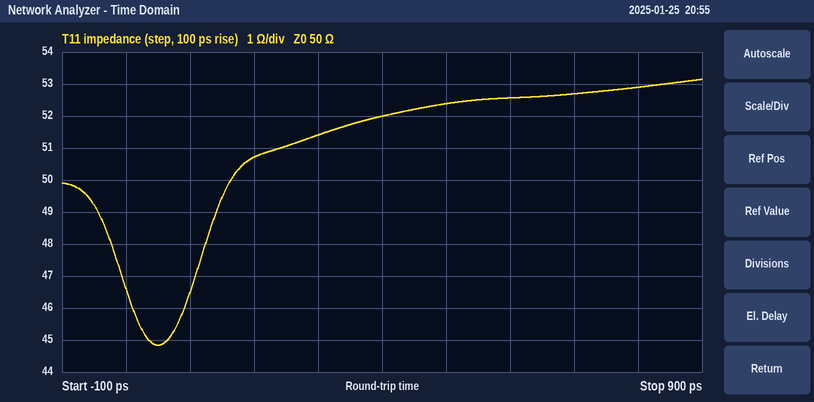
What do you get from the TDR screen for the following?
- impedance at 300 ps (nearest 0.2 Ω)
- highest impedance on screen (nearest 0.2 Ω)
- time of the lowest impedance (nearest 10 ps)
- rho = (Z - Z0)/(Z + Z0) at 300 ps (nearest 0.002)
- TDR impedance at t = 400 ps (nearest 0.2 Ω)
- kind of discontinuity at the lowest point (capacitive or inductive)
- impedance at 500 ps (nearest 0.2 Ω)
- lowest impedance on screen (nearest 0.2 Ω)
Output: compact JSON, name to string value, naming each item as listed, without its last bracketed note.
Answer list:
{"impedance at 300 ps": "51.4 Ω", "highest impedance on screen": "53.2 Ω", "time of the lowest impedance": "50 ps", "rho = (Z - Z0)/(Z + Z0) at 300 ps": "+0.014", "TDR impedance at t = 400 ps": "52.0 Ω", "kind of discontinuity at the lowest point": "capacitive", "impedance at 500 ps": "52.4 Ω", "lowest impedance on screen": "44.8 Ω"}
